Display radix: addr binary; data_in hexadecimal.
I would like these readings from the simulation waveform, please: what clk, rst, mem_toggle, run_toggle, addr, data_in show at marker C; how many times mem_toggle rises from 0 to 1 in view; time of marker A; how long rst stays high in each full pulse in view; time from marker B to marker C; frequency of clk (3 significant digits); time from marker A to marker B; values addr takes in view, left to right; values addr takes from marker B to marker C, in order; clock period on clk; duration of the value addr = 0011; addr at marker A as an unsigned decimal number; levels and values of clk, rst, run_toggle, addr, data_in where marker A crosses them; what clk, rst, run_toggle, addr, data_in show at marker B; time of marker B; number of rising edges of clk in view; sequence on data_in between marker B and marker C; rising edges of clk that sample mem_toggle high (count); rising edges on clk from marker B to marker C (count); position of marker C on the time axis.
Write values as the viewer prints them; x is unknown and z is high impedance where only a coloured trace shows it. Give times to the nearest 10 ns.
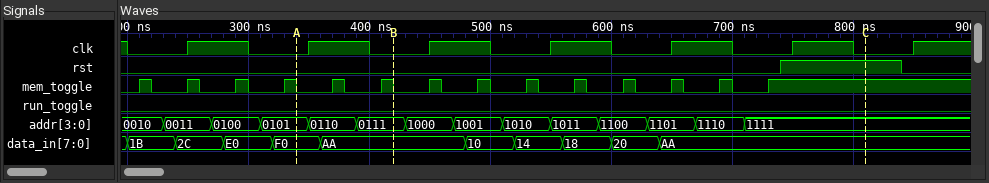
clk=0, rst=1, mem_toggle=1, run_toggle=0, addr=1111, data_in=AA
14
340 ns
100 ns
390 ns
10.0 MHz
80 ns
0010, 0011, 0100, 0101, 0110, 0111, 1000, 1001, 1010, 1011, 1100, 1101, 1110, 1111
0111, 1000, 1001, 1010, 1011, 1100, 1101, 1110, 1111
100 ns
40 ns
5
clk=0, rst=0, run_toggle=0, addr=0101, data_in=F0
clk=0, rst=0, run_toggle=0, addr=0111, data_in=AA
420 ns
7
AA, 10, 14, 18, 20, AA
2
4
810 ns
